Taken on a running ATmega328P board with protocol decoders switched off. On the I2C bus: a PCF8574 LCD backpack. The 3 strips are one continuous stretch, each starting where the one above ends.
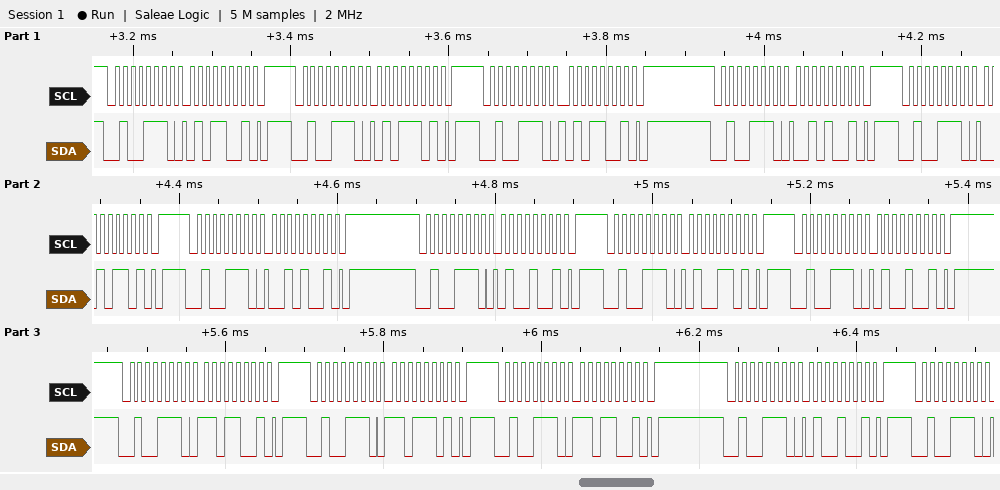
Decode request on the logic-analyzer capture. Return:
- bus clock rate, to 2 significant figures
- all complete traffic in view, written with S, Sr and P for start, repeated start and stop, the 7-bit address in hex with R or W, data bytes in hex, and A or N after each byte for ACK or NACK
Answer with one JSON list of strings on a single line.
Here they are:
["100 kHz", "S 27W A 59 A P S 27W A 5D A P S 27W A 59 A P S 27W A 29 A P S 27W A 2D A P S 27W A 29 A P S 27W A 49 A P S 27W A 4D A P S 27W A 49 A P S 27W A D9 A P S 27W A DD A P S 27W A D9 A P S 27W A 49 A P S 27W A"]
